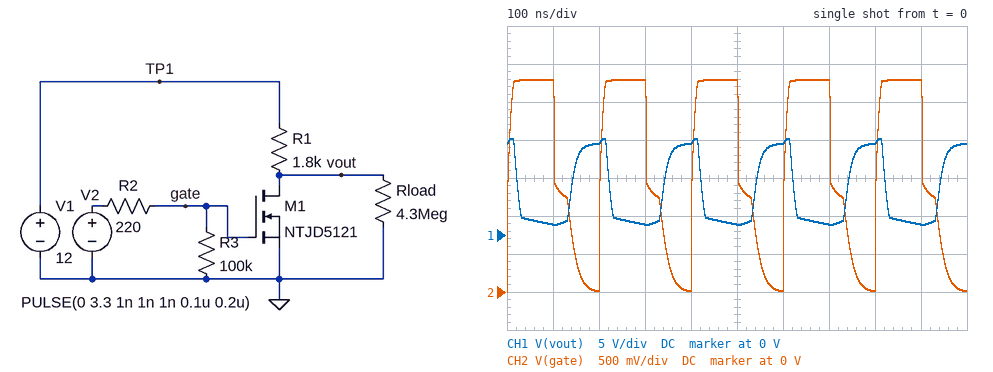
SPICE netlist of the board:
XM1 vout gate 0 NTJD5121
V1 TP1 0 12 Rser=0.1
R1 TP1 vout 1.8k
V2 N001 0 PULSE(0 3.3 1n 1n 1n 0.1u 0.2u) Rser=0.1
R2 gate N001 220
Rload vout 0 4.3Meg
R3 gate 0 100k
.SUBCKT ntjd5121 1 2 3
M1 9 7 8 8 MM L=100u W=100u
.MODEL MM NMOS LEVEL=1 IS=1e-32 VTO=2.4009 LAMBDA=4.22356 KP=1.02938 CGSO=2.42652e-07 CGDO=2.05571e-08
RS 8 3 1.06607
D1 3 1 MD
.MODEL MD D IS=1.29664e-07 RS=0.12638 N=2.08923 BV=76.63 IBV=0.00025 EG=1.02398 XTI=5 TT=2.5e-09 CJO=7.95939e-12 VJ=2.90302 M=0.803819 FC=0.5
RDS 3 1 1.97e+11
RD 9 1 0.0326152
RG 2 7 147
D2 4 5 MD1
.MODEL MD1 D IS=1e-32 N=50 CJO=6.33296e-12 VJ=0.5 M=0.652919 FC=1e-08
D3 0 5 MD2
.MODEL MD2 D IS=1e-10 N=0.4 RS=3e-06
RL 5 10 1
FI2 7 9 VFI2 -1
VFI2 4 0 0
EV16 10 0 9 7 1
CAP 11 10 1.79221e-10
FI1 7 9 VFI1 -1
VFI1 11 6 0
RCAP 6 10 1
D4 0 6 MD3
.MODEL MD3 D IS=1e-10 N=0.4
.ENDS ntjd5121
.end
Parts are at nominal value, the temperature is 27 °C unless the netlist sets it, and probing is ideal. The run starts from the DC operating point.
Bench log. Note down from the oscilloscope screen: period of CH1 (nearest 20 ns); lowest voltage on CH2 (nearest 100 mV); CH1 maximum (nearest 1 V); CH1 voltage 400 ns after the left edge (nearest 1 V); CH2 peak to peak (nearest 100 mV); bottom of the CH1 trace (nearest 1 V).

200 ns
0 V
13 V
12 V
2.8 V
1 V
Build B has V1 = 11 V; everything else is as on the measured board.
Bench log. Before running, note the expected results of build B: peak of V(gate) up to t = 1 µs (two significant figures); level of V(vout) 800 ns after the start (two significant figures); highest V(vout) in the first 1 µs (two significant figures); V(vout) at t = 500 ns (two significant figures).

2.8 V
11 V
12 V
1.3 V
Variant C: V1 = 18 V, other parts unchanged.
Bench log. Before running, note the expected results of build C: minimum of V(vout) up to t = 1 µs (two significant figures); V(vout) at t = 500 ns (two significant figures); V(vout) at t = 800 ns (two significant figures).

1.4 V
1.5 V
18 V
